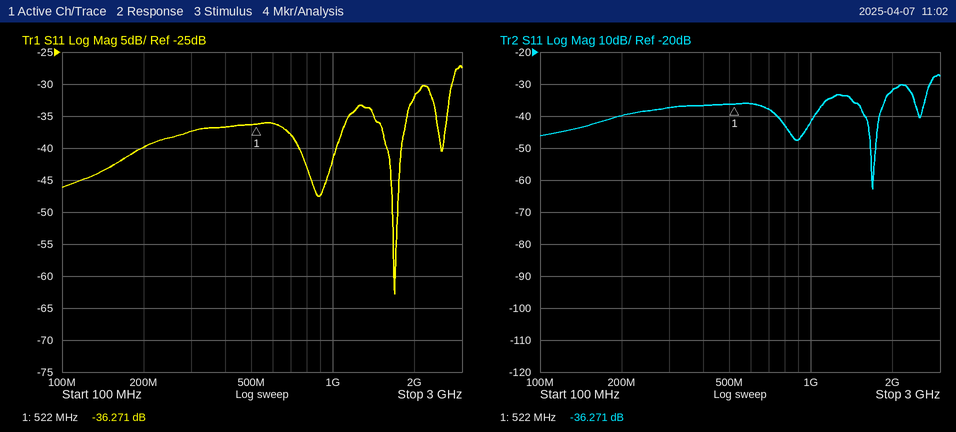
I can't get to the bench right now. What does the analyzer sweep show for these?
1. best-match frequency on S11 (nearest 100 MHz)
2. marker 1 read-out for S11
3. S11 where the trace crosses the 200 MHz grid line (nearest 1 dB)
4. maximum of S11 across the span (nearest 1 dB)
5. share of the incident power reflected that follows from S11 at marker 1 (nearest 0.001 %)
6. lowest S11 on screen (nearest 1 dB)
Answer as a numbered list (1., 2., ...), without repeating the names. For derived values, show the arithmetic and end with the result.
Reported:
1. 1.7 GHz
2. -36.271 dB
3. -40 dB
4. -27 dB
5. 10^(-36.271/10) ≈ 0.024 %
6. -63 dB
